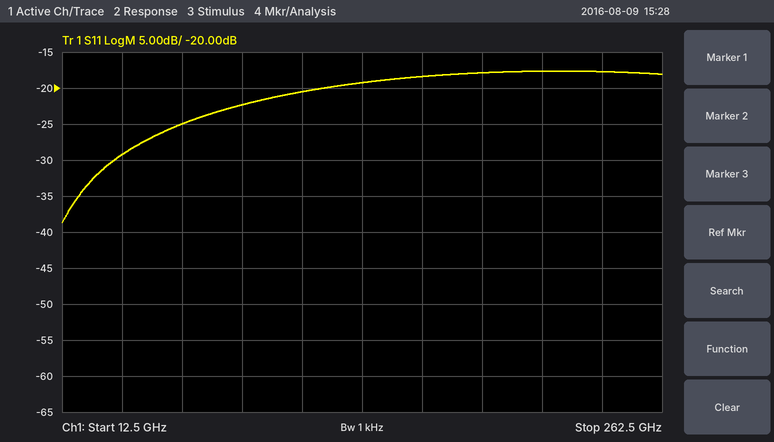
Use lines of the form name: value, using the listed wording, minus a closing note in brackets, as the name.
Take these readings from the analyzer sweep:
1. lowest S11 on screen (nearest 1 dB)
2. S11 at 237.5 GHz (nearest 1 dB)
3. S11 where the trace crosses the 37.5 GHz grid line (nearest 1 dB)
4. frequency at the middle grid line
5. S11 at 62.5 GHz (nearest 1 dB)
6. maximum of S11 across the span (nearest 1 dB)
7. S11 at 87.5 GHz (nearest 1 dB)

lowest S11 on screen: -39 dB
S11 at 237.5 GHz: -18 dB
S11 where the trace crosses the 37.5 GHz grid line: -29 dB
frequency at the middle grid line: 137.5 GHz
S11 at 62.5 GHz: -25 dB
maximum of S11 across the span: -18 dB
S11 at 87.5 GHz: -22 dB
